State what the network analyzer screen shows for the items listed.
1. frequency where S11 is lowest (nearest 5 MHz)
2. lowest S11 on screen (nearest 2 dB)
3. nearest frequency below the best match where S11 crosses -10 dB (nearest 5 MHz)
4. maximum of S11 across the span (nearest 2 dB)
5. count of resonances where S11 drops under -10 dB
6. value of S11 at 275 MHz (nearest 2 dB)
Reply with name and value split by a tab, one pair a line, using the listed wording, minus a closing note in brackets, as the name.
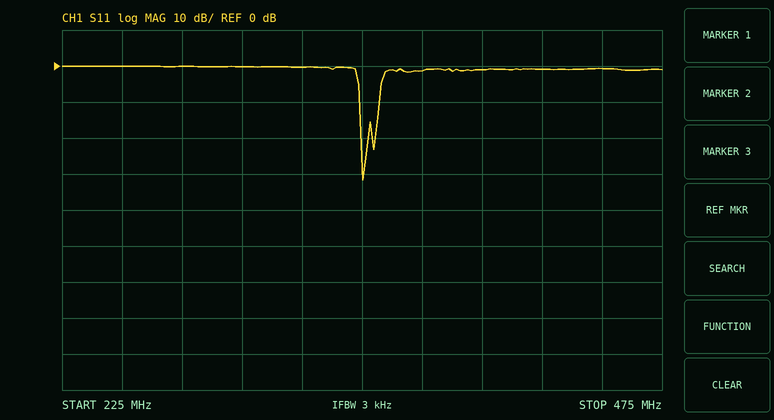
frequency where S11 is lowest	350 MHz
lowest S11 on screen	-32 dB
nearest frequency below the best match where S11 crosses -10 dB	350 MHz
maximum of S11 across the span	0 dB
count of resonances where S11 drops under -10 dB	2
value of S11 at 275 MHz	0 dB
